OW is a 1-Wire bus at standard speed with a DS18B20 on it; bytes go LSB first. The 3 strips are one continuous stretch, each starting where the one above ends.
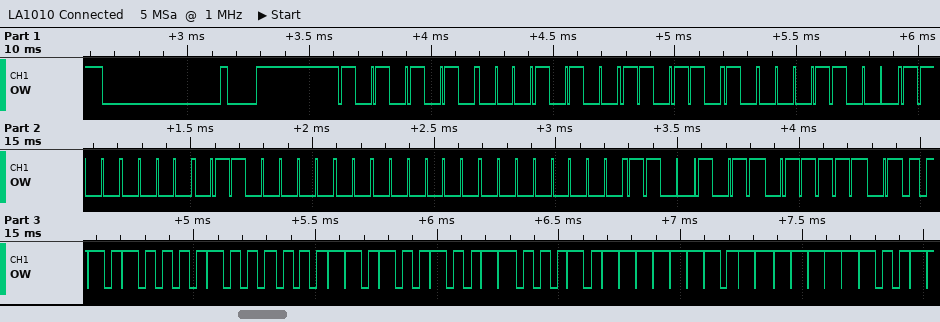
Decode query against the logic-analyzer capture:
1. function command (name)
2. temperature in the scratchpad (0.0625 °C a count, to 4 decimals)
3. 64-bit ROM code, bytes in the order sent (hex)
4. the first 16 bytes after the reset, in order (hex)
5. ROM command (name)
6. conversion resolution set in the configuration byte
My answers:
Read Scratchpad
33.2500 °C
28 5B 18 03 06 00 00 D3
55 28 5B 18 03 06 00 00 D3 BE 14 02 4B 46 7F FF
Match ROM
12 bits
